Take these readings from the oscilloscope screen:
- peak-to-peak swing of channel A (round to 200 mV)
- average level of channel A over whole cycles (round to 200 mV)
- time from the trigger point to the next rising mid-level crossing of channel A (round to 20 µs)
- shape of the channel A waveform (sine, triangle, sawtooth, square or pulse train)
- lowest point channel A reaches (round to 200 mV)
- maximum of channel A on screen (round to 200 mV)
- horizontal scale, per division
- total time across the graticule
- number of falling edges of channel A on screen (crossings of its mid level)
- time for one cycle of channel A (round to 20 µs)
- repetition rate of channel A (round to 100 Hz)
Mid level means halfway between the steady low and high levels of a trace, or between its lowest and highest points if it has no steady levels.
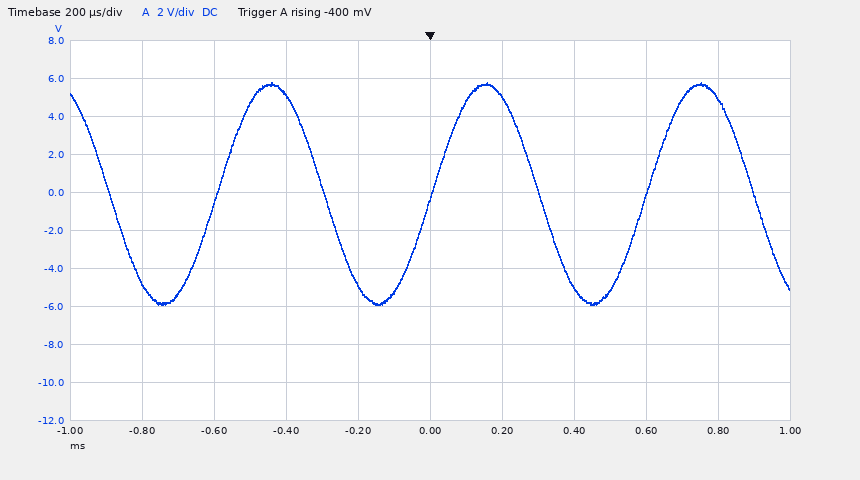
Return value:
11.6 V
0.0 V
600 µs
sine
-5.8 V
5.8 V
200 µs
2 ms
4
600 µs
1.7 kHz
